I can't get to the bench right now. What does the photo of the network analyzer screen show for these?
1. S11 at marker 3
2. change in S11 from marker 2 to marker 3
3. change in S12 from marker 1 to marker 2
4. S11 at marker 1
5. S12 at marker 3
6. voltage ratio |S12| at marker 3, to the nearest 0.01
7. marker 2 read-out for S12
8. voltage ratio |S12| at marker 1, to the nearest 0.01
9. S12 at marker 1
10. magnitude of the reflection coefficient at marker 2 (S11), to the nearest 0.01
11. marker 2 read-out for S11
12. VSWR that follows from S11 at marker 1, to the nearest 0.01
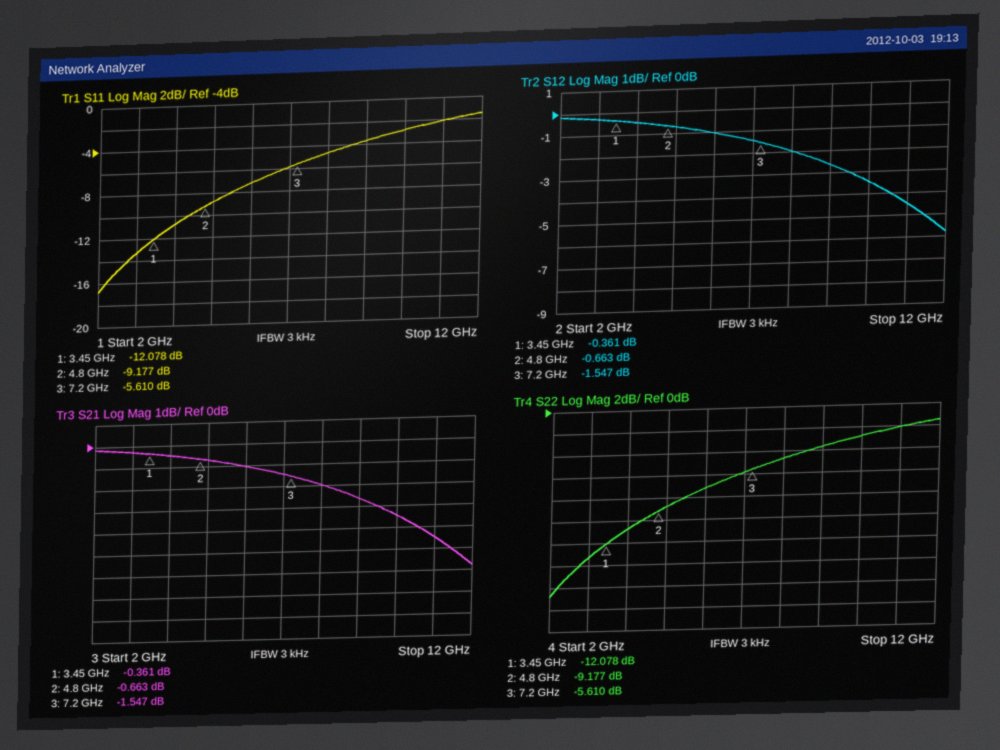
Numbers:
-5.610 dB
3.567 dB
-0.302 dB
-12.078 dB
-1.547 dB
0.84
-0.663 dB
0.96
-0.361 dB
0.35
-9.177 dB
1.66
